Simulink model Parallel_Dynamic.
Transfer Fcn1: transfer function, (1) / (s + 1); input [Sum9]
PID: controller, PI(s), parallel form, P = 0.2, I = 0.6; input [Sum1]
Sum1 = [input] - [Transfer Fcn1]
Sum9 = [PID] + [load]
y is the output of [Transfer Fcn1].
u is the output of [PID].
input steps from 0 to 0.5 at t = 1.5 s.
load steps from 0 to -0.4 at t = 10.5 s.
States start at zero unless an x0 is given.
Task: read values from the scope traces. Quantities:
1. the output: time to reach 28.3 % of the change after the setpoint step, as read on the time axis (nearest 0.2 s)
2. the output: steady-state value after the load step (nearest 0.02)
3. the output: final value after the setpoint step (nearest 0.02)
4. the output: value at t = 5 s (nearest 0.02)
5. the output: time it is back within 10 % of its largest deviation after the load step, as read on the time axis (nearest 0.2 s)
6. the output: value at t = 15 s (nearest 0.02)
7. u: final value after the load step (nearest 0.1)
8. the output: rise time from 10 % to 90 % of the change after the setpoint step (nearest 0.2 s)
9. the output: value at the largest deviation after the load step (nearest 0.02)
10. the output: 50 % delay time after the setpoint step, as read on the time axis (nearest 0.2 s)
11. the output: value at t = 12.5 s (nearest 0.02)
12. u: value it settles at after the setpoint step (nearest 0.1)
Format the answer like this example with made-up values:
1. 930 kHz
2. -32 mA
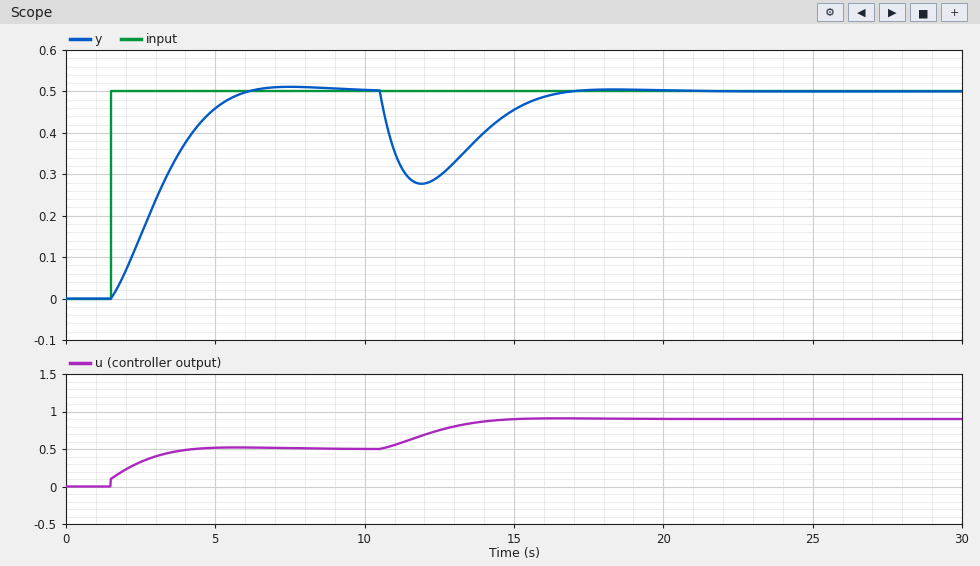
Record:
1. 2.4 s
2. 0.50
3. 0.50
4. 0.46
5. 15.6 s
6. 0.46
7. 0.9
8. 3.0 s
9. 0.28
10. 3.0 s
11. 0.30
12. 0.5
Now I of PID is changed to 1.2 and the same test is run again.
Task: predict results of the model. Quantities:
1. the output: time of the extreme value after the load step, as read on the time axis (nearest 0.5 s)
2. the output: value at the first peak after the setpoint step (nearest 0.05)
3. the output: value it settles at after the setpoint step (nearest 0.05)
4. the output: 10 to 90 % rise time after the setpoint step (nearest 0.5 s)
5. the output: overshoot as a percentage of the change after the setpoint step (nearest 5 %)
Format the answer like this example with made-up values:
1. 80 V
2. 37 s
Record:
1. 11.5 s
2. 0.55
3. 0.50
4. 1.5 s
5. 15 %
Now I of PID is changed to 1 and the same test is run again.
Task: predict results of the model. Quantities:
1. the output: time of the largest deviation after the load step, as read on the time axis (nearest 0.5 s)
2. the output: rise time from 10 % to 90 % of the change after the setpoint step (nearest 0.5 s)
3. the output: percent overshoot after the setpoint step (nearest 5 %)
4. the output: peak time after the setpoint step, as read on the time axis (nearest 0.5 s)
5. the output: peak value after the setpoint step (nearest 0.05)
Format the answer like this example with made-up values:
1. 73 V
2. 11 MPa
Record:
1. 11.5 s
2. 2.0 s
3. 10 %
4. 5.0 s
5. 0.55
